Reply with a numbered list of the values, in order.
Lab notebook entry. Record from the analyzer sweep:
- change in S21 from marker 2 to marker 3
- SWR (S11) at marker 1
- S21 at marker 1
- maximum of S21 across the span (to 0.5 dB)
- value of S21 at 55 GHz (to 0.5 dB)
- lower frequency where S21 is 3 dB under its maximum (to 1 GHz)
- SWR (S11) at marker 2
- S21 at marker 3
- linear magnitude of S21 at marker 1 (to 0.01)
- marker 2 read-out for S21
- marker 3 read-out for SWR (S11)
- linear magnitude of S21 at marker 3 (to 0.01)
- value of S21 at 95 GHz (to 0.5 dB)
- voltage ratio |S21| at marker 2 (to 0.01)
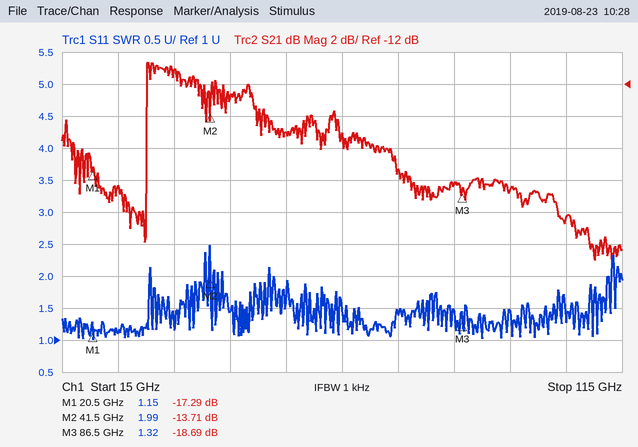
1. -4.98 dB
2. 1.15
3. -17.29 dB
4. -10.5 dB
5. -15.0 dB
6. 30 GHz
7. 1.99
8. -18.69 dB
9. 0.14
10. -13.71 dB
11. 1.32
12. 0.12
13. -18.5 dB
14. 0.21
